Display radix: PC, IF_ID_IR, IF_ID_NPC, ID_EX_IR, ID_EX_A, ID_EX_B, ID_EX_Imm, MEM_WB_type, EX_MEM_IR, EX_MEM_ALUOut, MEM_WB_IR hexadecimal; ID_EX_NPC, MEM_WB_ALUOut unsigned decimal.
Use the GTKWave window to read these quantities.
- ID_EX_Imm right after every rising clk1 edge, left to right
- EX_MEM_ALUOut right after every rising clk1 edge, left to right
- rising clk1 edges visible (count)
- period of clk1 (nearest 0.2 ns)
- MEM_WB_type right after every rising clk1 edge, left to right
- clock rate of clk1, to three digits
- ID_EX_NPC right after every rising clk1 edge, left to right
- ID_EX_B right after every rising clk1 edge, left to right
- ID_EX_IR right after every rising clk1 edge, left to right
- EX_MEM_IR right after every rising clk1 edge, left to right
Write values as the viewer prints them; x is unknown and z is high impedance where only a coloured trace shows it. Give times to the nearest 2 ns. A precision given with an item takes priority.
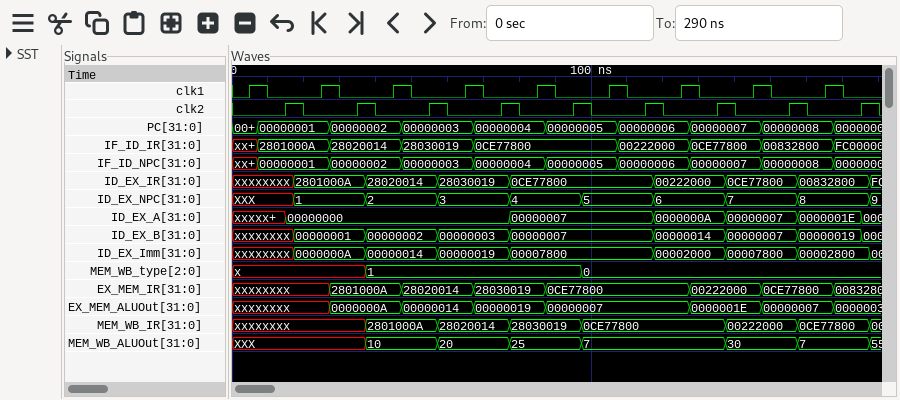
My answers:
xxxxxxxx, 0000000A, 00000014, 00000019, 00007800, 00007800, 00002000, 00007800, 00002800
xxxxxxxx, xxxxxxxx, 0000000A, 00000014, 00000019, 00000007, 00000007, 0000001E, 00000007
9
20 ns
x, x, 1, 1, 1, 0, 0, 0, 0
50.0 MHz
XXX, 1, 2, 3, 4, 5, 6, 7, 8
xxxxxxxx, 00000001, 00000002, 00000003, 00000007, 00000007, 00000014, 00000007, 00000019
xxxxxxxx, 2801000A, 28020014, 28030019, 0CE77800, 0CE77800, 00222000, 0CE77800, 00832800
xxxxxxxx, xxxxxxxx, 2801000A, 28020014, 28030019, 0CE77800, 0CE77800, 00222000, 0CE77800
